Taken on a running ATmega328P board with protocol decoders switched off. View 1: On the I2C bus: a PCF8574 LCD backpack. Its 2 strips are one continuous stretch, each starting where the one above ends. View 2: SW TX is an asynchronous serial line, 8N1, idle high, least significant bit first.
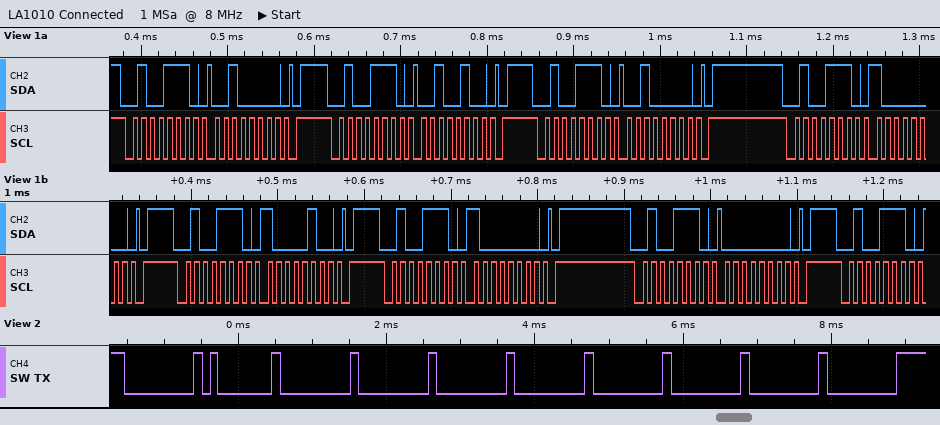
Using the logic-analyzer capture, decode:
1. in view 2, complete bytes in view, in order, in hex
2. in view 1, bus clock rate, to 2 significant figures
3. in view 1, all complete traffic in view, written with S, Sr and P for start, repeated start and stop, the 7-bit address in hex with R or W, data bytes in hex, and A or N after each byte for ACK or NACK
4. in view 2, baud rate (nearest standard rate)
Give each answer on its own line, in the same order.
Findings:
00 01 00 00 00 00 00 00 00 00
100 kHz
S 27W A 20 A P S 27W A 24 A P S 27W A 20 A P S 27W A 80 A P S 27W A 84 A P S 27W A 80 A P S 27W A 00 A P S 27W A
9600 baud
